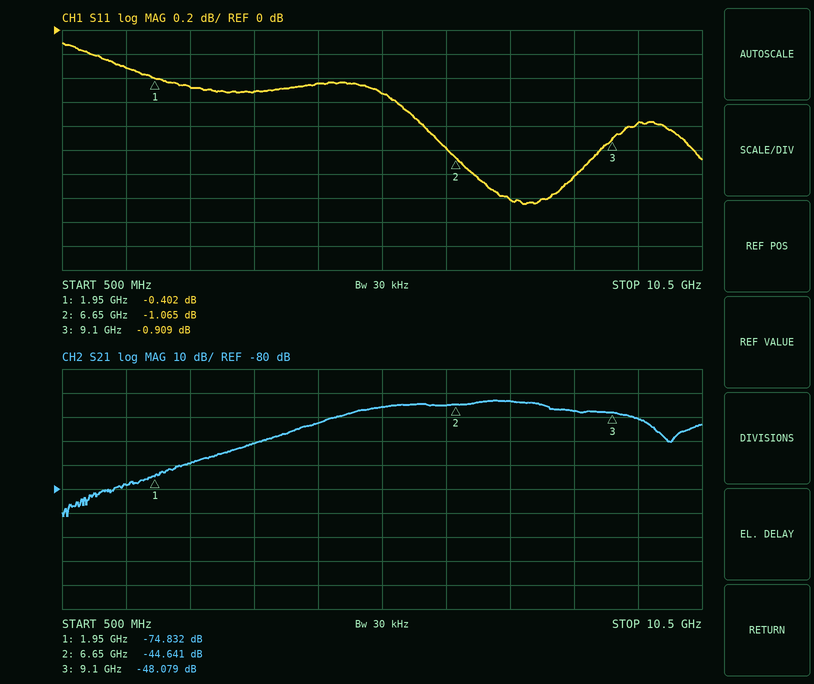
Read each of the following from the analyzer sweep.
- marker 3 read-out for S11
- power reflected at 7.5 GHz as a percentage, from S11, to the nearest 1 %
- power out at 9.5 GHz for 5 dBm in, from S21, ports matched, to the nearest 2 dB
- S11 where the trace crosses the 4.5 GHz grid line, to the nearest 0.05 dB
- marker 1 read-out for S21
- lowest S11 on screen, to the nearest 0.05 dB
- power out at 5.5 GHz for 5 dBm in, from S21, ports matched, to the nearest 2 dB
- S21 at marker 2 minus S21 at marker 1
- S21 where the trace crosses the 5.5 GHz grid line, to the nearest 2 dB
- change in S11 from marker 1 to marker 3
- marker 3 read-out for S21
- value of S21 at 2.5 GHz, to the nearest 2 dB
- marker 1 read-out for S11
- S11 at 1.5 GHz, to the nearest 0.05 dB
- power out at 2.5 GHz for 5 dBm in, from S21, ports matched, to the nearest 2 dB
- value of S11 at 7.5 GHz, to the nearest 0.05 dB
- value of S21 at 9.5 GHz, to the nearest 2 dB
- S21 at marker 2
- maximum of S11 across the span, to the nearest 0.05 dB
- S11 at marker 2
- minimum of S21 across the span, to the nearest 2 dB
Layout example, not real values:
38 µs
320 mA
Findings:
-0.909 dB
72 %
-46 dBm
-0.45 dB
-74.832 dB
-1.45 dB
-40 dBm
30.191 dB
-46 dB
-0.507 dB
-48.079 dB
-70 dB
-0.402 dB
-0.30 dB
-64 dBm
-1.40 dB
-50 dB
-44.641 dB
-0.10 dB
-1.065 dB
-92 dB
